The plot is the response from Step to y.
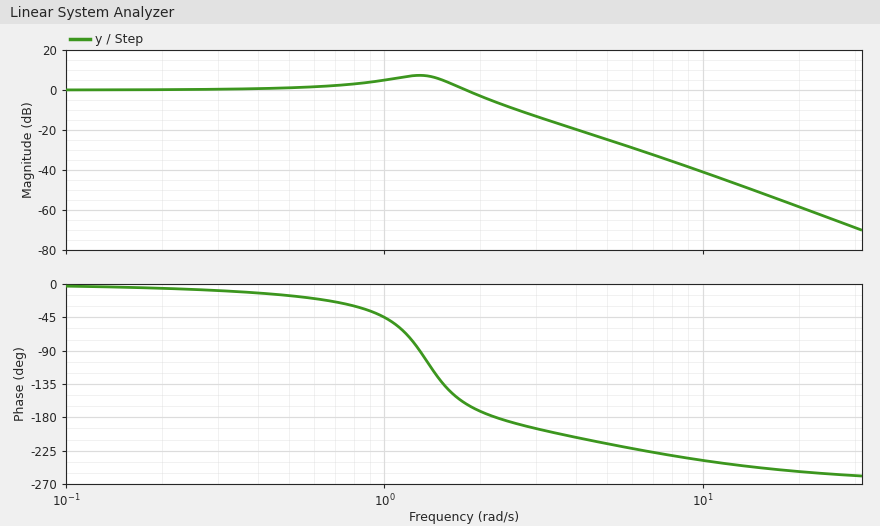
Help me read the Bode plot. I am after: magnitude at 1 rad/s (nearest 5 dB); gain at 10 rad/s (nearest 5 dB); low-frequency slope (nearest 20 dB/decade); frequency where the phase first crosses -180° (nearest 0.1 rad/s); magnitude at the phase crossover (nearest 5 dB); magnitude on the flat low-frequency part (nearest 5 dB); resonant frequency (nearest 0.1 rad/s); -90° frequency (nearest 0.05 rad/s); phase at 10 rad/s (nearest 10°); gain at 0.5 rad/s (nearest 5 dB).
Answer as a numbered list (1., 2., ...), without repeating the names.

1. 5 dB
2. -40 dB
3. 0 dB/decade
4. 2.2 rad/s
5. -5 dB
6. 0 dB
7. 1.3 rad/s
8. 1.30 rad/s
9. -240°
10. 0 dB
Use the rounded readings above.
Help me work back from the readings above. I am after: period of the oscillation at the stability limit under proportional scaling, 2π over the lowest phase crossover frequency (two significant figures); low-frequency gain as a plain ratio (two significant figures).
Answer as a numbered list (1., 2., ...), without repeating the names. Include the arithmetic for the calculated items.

1. 2π / 2.2 = 2.9 s
2. 10^(0 / 20) = 1.0
